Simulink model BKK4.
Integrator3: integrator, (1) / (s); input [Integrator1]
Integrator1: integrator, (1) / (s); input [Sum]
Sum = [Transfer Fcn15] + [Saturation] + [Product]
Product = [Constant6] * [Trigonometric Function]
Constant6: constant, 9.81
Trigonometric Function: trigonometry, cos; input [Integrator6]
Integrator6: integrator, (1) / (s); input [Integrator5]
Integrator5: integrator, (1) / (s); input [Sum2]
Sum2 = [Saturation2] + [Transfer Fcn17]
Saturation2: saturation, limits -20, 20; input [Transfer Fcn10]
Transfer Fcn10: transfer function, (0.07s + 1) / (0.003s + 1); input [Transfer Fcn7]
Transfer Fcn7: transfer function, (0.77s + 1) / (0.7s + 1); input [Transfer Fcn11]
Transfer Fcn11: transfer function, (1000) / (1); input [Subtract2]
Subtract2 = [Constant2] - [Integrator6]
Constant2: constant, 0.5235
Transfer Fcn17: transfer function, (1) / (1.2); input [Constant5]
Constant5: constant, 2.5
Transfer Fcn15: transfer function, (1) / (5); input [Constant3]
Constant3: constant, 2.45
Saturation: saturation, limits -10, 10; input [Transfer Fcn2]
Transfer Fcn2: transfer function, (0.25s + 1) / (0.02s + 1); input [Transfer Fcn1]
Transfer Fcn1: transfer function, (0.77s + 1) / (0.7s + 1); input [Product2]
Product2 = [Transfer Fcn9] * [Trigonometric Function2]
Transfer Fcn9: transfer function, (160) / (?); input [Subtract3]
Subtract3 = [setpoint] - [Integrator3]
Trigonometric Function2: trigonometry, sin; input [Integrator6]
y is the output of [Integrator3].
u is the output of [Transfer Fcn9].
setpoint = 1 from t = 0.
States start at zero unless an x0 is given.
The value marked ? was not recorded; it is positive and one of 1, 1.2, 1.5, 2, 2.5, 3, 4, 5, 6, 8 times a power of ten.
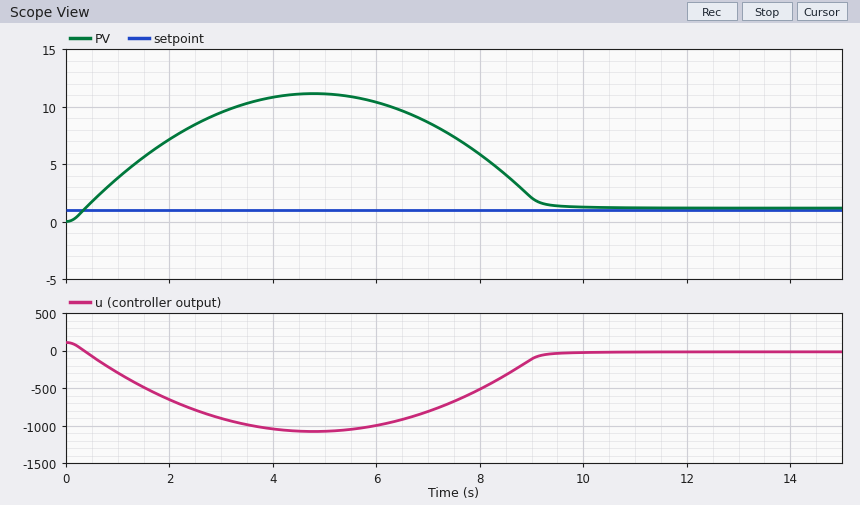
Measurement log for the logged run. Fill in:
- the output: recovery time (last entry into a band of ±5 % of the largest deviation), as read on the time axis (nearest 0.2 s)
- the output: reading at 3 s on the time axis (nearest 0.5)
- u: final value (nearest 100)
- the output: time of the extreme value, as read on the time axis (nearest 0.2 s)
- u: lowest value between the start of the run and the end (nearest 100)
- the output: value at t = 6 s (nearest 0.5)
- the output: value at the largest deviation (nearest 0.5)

9.2 s
9.5
0
4.8 s
-1100
10.5
11.0
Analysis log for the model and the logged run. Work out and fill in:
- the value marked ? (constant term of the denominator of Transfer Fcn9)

1.5
